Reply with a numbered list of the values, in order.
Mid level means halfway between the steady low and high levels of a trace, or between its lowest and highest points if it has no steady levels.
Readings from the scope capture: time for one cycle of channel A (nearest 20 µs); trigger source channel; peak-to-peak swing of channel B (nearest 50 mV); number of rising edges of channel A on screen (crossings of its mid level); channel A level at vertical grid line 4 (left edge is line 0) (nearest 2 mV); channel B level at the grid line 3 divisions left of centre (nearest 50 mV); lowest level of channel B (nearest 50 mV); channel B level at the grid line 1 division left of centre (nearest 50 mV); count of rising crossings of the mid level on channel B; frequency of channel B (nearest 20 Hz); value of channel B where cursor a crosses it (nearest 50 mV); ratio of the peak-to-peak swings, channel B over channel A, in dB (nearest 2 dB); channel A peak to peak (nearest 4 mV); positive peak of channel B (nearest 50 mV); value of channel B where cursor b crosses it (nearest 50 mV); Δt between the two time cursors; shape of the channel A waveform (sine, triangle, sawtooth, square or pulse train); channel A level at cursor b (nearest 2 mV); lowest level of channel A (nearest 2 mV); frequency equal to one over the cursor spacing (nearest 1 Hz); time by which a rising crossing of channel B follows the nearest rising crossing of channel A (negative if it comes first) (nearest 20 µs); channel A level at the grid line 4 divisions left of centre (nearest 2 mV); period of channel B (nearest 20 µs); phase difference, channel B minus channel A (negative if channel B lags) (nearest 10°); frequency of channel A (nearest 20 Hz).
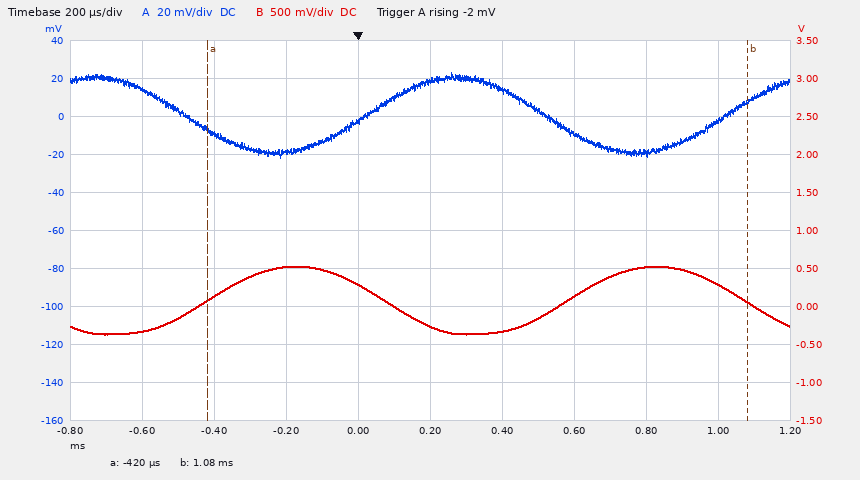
1. 1.00 ms
2. channel A
3. 900 mV
4. 2
5. -2 mV
6. 150 mV
7. -350 mV
8. 300 mV
9. 2
10. 1.00 kHz
11. 100 mV
12. 26 dB
13. 44 mV
14. 550 mV
15. 50 mV
16. 1.50 ms
17. sine
18. 8 mV
19. -22 mV
20. 667 Hz
21. -440 µs
22. 14 mV
23. 1.00 ms
24. +160°
25. 1.00 kHz
